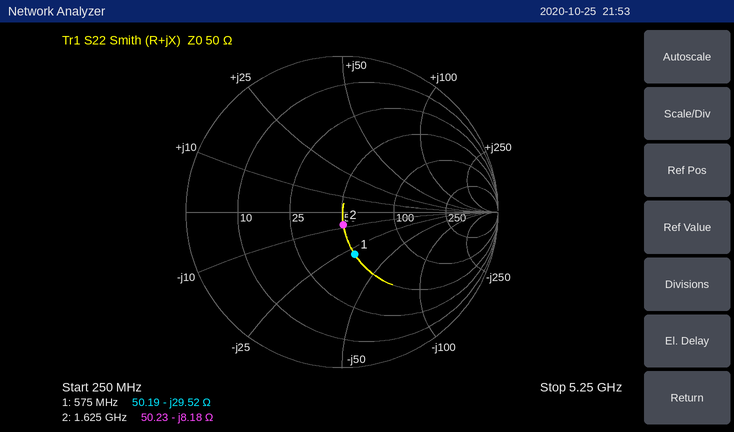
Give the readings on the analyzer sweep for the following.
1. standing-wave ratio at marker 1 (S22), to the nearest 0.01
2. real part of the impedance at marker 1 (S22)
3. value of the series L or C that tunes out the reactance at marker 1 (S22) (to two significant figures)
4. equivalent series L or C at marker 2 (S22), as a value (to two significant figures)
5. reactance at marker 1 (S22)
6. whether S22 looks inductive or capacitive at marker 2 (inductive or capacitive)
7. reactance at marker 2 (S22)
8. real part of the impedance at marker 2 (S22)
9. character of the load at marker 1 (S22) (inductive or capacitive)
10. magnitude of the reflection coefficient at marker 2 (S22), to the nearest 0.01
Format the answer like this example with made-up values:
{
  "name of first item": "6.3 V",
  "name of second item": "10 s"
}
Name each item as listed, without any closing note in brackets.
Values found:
{
  "standing-wave ratio at marker 1 (S22), to the nearest 0.01": "1.79",
  "real part of the impedance at marker 1": "50.19 Ω",
  "value of the series L or C that tunes out the reactance at marker 1 (S22)": "8.2 nH",
  "equivalent series L or C at marker 2 (S22), as a value": "12 pF",
  "reactance at marker 1": "-29.52 Ω",
  "whether S22 looks inductive or capacitive at marker 2": "capacitive",
  "reactance at marker 2": "-8.18 Ω",
  "real part of the impedance at marker 2": "50.23 Ω",
  "character of the load at marker 1 (S22)": "capacitive",
  "magnitude of the reflection coefficient at marker 2 (S22), to the nearest 0.01": "0.08"
}
